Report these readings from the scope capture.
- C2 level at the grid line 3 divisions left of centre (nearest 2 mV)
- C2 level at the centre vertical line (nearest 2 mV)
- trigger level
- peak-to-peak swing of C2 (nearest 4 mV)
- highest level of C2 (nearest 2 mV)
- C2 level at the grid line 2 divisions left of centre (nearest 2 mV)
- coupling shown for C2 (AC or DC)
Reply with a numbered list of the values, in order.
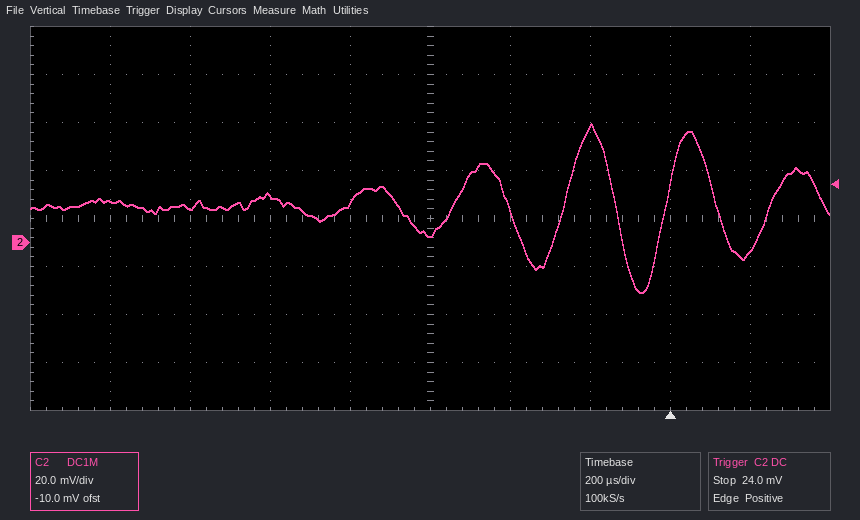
1. 14 mV
2. 4 mV
3. 24.0 mV
4. 72 mV
5. 50 mV
6. 20 mV
7. DC
